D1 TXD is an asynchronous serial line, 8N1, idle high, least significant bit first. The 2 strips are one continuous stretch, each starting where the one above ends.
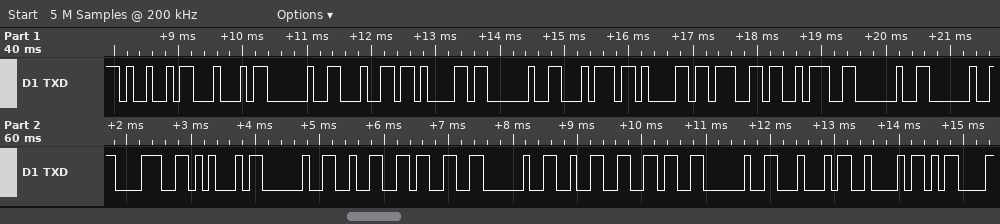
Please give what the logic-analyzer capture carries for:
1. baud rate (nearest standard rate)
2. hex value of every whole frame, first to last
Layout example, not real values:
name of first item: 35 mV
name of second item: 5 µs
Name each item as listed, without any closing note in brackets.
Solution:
baud rate: 9600 baud
hex value of every whole frame, first to last: 49 44 20 64 61 20 74 61 67 3A 20 20 38 45 20 32 33 20 32 36 20 44 42 0D
